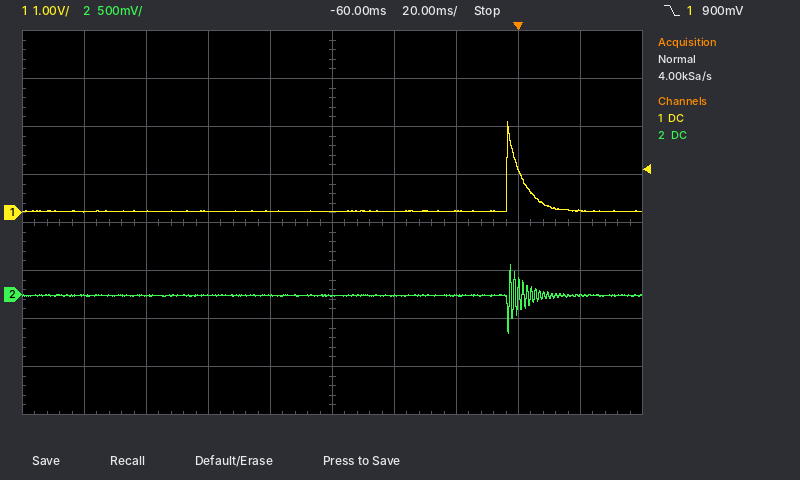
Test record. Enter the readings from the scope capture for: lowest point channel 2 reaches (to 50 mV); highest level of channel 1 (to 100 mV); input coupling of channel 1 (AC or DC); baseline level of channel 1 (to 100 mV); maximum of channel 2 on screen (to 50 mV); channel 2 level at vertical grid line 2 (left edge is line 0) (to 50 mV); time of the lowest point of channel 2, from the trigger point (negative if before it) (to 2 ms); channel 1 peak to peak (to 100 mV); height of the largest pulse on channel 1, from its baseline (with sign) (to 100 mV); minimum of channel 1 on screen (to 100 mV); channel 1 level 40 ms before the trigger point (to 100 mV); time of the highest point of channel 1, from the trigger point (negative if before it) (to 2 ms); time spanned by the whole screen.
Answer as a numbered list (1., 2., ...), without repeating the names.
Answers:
1. -400 mV
2. 1.9 V
3. DC
4. 0.0 V
5. 300 mV
6. 0 mV
7. -4 ms
8. 1.9 V
9. +1.9 V
10. 0.0 V
11. 0.0 V
12. -4 ms
13. 200 ms
